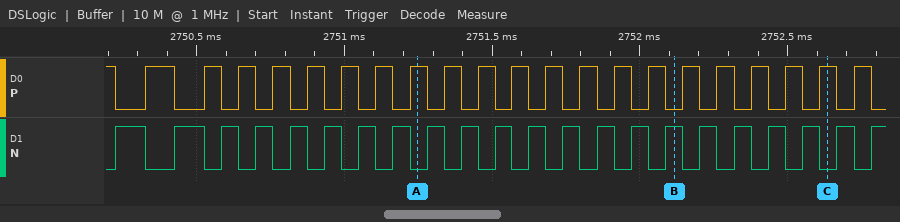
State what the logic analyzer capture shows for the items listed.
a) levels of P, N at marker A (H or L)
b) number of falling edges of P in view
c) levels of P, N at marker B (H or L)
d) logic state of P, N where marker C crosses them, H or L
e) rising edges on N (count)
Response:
P=H, N=L
22
P=L, N=H
P=H, N=L
22
